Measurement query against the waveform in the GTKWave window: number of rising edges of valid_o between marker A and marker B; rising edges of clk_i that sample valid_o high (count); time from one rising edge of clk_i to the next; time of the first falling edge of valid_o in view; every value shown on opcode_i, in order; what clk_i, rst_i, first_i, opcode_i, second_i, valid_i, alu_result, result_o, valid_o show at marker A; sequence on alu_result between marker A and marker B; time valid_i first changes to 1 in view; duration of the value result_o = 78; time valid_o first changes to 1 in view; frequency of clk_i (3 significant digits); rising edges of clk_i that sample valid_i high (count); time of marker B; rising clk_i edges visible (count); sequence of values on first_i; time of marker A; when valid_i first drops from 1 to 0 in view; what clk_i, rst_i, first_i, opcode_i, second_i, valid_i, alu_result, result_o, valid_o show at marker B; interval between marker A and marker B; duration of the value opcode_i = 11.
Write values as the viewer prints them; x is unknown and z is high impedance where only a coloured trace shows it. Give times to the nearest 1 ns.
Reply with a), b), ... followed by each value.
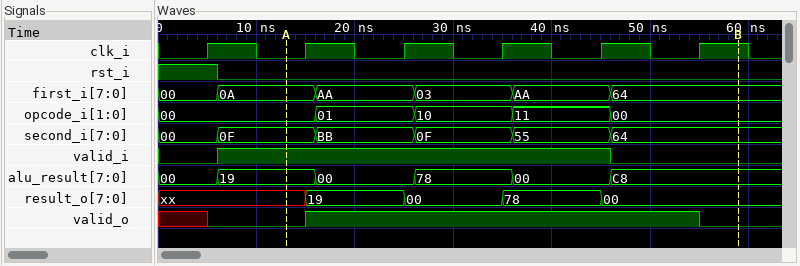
a) 1
b) 4
c) 10 ns
d) 55 ns
e) 00, 01, 10, 11, 00
f) clk_i=0, rst_i=0, first_i=0A, opcode_i=00, second_i=0F, valid_i=1, alu_result=19, result_o=xx, valid_o=0
g) 19, 00, 78, 00, C8
h) 6 ns
i) 10 ns
j) 15 ns
k) 100 MHz
l) 4
m) 59 ns
n) 6
o) 00, 0A, AA, 03, AA, 64
p) 13 ns
q) 46 ns
r) clk_i=1, rst_i=0, first_i=64, opcode_i=00, second_i=64, valid_i=0, alu_result=C8, result_o=00, valid_o=0
s) 46 ns
t) 10 ns
